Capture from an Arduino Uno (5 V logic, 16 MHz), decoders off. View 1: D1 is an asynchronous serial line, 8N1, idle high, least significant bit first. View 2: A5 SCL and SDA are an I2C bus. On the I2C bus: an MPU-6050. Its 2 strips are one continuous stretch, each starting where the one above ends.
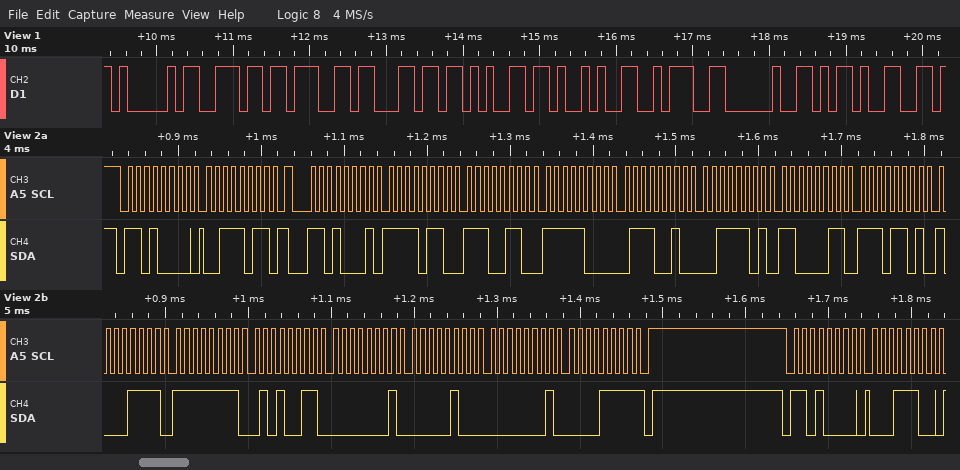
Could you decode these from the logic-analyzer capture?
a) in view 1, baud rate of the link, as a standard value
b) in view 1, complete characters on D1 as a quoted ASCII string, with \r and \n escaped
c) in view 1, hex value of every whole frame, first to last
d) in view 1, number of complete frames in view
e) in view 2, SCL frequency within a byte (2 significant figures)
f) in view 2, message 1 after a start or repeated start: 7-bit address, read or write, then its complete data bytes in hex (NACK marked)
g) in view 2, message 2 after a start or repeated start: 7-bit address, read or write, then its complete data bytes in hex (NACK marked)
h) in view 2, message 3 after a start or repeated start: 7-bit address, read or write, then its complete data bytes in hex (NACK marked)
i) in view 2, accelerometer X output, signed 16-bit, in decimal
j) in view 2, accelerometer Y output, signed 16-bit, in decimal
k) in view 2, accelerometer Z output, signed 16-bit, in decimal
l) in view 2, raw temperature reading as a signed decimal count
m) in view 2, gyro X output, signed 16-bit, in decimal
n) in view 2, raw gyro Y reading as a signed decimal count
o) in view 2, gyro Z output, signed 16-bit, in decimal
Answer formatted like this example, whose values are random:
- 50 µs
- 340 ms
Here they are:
- 9600 baud
- "Angle): -"
- 41 6E 67 6C 65 29 3A 20 2D
- 9
- 100 kHz
- 0x68 write: 3B
- 0x68 read: F6 E6 F8 72 3D C3 ED 8F FF 53 01 04 01 0F NACK
- 0x68 write: 1C
- -2330
- -1934
- 15811
- -4721
- -173
- 260
- 271
